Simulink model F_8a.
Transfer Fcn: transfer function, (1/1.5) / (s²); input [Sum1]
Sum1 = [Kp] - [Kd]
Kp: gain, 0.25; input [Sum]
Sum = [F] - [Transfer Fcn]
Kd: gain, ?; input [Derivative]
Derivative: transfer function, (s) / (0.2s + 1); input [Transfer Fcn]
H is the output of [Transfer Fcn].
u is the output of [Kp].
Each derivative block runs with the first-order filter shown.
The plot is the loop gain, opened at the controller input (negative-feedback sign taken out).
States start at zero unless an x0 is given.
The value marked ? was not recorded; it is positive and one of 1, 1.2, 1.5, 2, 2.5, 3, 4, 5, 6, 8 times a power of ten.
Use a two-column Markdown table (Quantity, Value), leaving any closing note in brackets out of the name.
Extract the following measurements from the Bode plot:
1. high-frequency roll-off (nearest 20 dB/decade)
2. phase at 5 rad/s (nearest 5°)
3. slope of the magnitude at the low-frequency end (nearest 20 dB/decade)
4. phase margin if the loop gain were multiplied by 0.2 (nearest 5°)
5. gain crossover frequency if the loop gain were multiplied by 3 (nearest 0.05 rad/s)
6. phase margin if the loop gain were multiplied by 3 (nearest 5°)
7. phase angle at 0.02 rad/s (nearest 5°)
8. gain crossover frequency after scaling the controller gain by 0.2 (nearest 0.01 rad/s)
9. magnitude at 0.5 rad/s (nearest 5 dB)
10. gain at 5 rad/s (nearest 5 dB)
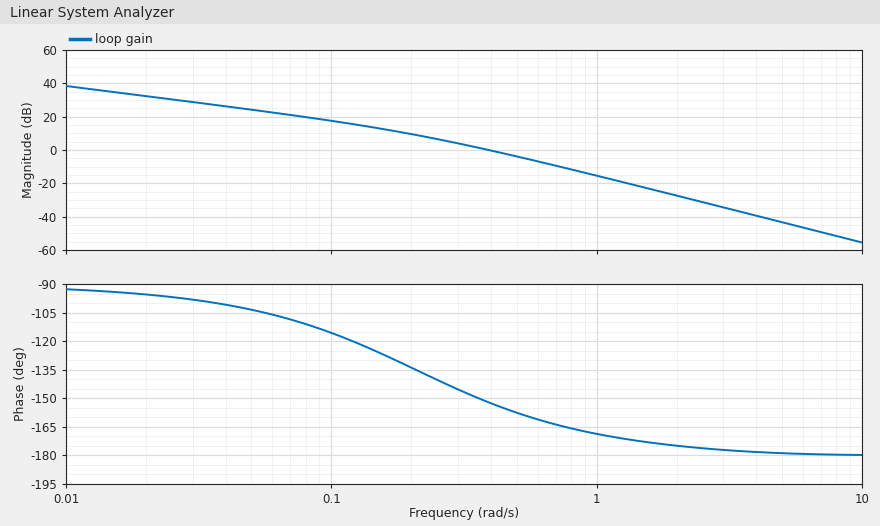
| Quantity | Value |
|---|---|
| high-frequency roll-off | -40 dB/decade |
| phase at 5 rad/s | -180° |
| slope of the magnitude at the low-frequency end | -20 dB/decade |
| phase margin if the loop gain were multiplied by 0.2 | 55° |
| gain crossover frequency if the loop gain were multiplied by 3 | 0.70 rad/s |
| phase margin if the loop gain were multiplied by 3 | 15° |
| phase angle at 0.02 rad/s | -95° |
| gain crossover frequency after scaling the controller gain by 0.2 | 0.14 rad/s |
| magnitude at 0.5 rad/s | -5 dB |
| gain at 5 rad/s | -45 dB |
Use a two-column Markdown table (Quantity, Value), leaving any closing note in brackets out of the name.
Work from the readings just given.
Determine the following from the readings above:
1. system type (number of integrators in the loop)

| Quantity | Value |
|---|---|
| system type | 1 |
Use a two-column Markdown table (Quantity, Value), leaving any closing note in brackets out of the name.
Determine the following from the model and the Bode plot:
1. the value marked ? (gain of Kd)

| Quantity | Value |
|---|---|
| the value marked ? | 0.3 |
